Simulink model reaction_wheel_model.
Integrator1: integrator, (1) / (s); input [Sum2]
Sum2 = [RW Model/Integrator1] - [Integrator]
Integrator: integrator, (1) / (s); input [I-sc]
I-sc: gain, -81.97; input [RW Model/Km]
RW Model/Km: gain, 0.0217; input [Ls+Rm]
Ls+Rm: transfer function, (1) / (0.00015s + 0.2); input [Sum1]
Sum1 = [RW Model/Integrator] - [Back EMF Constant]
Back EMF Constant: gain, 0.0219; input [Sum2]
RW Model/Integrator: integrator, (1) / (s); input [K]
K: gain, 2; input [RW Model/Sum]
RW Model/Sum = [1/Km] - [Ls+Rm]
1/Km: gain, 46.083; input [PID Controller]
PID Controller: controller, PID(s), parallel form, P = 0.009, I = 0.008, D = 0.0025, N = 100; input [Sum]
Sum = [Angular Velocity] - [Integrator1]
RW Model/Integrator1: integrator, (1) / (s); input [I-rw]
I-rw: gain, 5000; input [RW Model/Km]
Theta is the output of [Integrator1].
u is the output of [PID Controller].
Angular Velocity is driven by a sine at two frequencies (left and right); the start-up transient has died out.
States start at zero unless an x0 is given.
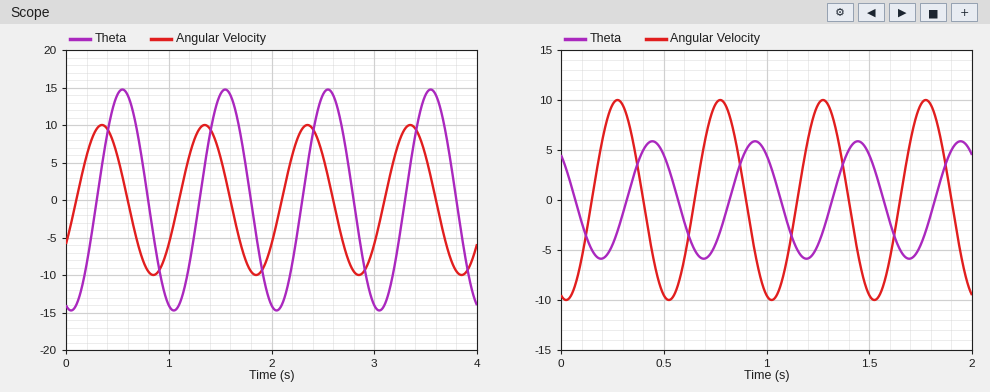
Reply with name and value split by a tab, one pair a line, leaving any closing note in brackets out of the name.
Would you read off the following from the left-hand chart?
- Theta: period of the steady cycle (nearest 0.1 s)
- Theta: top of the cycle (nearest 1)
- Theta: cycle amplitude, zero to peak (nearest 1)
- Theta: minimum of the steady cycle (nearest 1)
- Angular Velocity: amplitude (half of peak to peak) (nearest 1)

Theta: period of the steady cycle	1.0 s
Theta: top of the cycle	15
Theta: cycle amplitude, zero to peak	15
Theta: minimum of the steady cycle	-15
Angular Velocity: amplitude (half of peak to peak)	10
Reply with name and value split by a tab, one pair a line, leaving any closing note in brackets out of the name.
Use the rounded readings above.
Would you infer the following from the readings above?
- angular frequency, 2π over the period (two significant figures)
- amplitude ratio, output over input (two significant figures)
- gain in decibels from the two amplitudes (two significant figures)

angular frequency, 2π over the period	6.3 rad/s
amplitude ratio, output over input	1.5
gain in decibels from the two amplitudes	3.5 dB
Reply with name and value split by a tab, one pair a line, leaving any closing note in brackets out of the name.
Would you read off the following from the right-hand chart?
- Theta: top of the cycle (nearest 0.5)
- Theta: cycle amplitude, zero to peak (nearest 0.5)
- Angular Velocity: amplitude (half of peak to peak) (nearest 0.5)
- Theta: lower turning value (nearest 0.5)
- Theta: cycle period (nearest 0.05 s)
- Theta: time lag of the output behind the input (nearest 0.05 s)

Theta: top of the cycle	6.0
Theta: cycle amplitude, zero to peak	6.0
Angular Velocity: amplitude (half of peak to peak)	10.0
Theta: lower turning value	-6.0
Theta: cycle period	0.50 s
Theta: time lag of the output behind the input	0.15 s
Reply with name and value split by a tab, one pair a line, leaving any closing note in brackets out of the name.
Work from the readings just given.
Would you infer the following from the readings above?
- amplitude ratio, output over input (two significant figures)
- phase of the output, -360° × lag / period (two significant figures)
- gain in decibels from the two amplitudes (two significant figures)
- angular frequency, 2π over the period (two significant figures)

amplitude ratio, output over input	0.60
phase of the output, -360° × lag / period	-110°
gain in decibels from the two amplitudes	-4.4 dB
angular frequency, 2π over the period	13 rad/s
